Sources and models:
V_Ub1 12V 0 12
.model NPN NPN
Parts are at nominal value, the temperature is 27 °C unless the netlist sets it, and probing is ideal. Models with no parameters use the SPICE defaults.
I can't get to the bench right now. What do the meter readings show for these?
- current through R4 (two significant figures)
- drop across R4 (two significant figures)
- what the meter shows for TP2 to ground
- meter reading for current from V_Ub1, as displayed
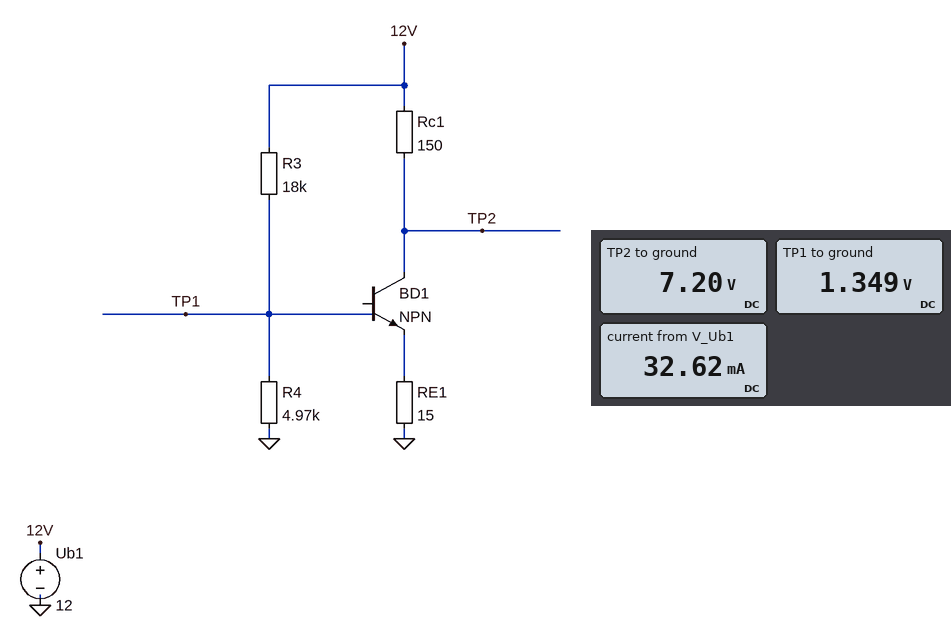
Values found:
270 µA
1.3 V
7.20 V
32.62 mA
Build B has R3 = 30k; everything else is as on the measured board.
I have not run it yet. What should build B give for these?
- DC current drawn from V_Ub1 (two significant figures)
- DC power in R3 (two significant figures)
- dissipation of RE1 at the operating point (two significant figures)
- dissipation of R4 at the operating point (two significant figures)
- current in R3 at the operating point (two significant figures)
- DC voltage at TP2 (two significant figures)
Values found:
15 mA
4.0 mW
3.4 mW
230 µW
360 µA
9.8 V
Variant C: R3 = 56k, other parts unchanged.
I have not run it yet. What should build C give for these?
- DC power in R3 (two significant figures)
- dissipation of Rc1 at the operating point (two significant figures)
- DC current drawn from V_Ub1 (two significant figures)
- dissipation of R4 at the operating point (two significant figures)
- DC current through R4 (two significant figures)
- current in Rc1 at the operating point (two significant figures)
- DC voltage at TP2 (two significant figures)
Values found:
2.2 mW
1.3 mW
3.1 mA
140 µW
170 µA
2.9 mA
12 V
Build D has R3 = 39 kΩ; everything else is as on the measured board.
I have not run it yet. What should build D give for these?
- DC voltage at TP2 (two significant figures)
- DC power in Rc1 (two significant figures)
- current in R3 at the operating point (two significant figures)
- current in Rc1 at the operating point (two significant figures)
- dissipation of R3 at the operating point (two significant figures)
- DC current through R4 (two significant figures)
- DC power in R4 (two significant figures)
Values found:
11 V
12 mW
280 µA
8.9 mA
3.1 mW
190 µA
190 µW
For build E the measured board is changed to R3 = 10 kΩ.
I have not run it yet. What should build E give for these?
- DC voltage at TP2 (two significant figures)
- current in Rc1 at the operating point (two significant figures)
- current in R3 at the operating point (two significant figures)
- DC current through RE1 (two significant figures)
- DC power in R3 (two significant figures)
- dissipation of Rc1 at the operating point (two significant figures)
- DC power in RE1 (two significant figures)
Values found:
2.4 V
64 mA
1.0 mA
65 mA
10 mW
620 mW
63 mW
